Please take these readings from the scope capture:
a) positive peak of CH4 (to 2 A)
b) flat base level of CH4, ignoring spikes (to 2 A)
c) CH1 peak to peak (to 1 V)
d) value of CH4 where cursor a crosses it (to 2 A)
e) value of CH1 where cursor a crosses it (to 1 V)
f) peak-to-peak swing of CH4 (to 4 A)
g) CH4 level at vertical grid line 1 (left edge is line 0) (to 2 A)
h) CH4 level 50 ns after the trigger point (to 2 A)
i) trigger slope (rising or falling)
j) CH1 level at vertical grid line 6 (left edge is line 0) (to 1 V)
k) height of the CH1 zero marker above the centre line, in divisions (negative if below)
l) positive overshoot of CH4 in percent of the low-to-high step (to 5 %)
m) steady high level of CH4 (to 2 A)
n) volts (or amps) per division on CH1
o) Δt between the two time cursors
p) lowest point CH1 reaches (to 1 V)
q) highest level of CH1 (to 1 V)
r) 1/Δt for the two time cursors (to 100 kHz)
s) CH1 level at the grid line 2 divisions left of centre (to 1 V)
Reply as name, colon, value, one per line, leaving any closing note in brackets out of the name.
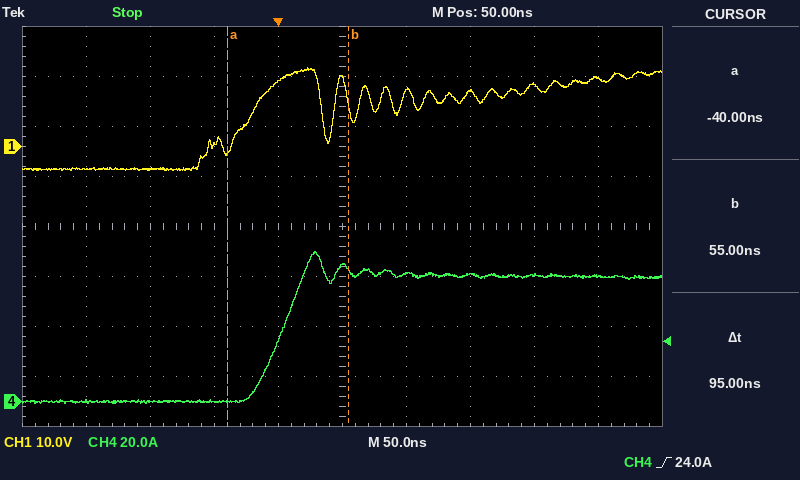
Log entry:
positive peak of CH4: 60 A
flat base level of CH4, ignoring spikes: 0 A
CH1 peak to peak: 21 V
value of CH4 where cursor a crosses it: 0 A
value of CH1 where cursor a crosses it: -1 V
peak-to-peak swing of CH4: 60 A
CH4 level at vertical grid line 1 (left edge is line 0): 0 A
CH4 level 50 ns after the trigger point: 54 A
trigger slope: rising
CH1 level at vertical grid line 6 (left edge is line 0): 11 V
height of the CH1 zero marker above the centre line, in divisions: +1.6 div
positive overshoot of CH4 in percent of the low-to-high step: 20 %
steady high level of CH4: 50 A
volts (or amps) per division on CH1: 10 V
Δt between the two time cursors: 95 ns
lowest point CH1 reaches: -5 V
highest level of CH1: 16 V
1/Δt for the two time cursors: 10.5 MHz
CH1 level at the grid line 2 divisions left of centre: 0 V
